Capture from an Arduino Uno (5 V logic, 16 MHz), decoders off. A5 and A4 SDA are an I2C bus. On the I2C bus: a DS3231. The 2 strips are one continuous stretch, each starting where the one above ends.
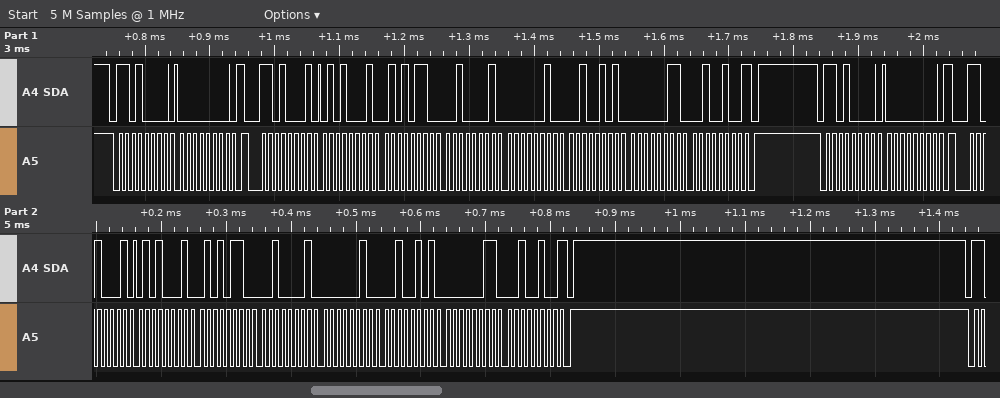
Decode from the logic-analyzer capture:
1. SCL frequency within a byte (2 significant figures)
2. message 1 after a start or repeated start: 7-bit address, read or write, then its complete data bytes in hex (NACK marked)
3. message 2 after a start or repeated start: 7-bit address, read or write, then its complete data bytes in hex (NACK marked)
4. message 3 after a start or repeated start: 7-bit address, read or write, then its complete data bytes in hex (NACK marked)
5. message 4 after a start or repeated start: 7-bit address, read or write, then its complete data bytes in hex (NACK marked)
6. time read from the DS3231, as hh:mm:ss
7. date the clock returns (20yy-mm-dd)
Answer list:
100 kHz
0x68 write: 00
0x68 read: 51 56 21 02 25 03 24 NACK
0x68 write: 00
0x68 read: 51 56 21 02 25 03 24 NACK
21:56:51
2024-03-25
